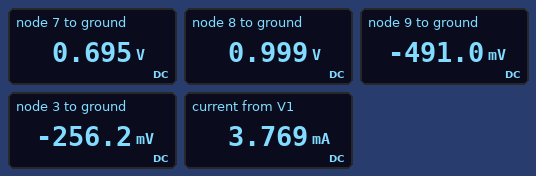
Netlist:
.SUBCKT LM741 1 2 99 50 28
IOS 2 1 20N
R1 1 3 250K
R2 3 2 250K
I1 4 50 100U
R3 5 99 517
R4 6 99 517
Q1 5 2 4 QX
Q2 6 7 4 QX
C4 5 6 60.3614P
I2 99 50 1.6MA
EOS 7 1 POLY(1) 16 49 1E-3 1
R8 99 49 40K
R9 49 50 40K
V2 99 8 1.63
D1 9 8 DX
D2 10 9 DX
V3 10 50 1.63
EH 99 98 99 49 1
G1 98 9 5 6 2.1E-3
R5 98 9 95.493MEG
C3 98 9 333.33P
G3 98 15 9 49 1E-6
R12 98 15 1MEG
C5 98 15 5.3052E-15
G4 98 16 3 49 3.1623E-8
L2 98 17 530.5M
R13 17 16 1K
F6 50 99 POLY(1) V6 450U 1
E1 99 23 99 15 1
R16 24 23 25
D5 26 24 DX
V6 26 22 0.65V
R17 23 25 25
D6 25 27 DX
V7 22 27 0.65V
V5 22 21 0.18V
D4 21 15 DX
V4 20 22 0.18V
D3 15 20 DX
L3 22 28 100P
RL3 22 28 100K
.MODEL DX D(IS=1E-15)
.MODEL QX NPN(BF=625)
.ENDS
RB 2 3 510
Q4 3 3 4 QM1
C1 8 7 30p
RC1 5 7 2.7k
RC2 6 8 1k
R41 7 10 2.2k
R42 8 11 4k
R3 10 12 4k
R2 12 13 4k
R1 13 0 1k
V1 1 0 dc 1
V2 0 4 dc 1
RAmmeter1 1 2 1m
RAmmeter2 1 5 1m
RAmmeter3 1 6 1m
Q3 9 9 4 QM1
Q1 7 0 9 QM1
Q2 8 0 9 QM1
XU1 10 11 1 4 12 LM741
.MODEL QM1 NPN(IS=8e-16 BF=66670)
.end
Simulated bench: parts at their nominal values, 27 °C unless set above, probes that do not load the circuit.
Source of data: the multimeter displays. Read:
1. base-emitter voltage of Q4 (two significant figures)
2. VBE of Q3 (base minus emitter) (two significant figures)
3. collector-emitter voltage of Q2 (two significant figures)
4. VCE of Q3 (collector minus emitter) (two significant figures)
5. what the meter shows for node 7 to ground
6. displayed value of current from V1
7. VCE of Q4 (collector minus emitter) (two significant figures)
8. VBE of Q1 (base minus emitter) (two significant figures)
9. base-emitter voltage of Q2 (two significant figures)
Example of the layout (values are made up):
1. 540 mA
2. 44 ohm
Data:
1. 740 mV
2. 510 mV
3. 1.5 V
4. 510 mV
5. 0.695 V
6. 3.769 mA
7. 740 mV
8. 490 mV
9. 490 mV
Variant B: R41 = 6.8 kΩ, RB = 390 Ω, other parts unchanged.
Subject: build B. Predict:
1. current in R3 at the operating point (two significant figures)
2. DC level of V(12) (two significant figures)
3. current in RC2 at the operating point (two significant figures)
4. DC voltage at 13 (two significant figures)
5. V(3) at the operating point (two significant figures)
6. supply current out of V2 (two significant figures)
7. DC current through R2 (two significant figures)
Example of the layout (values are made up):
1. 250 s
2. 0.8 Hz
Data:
1. 76 µA
2. -16 mV
3. 1.7 µA
4. -3.2 mV
5. -250 mV
6. 4.5 mA
7. 3.2 µA
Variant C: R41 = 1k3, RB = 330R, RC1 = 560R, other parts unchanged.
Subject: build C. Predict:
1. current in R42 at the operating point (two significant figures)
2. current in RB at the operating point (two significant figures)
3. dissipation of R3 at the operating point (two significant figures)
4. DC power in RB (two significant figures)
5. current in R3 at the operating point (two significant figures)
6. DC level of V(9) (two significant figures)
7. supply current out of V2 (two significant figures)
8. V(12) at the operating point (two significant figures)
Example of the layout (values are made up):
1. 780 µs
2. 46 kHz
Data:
1. 810 nA
2. 3.8 mA
3. 120 µW
4. 4.7 mW
5. 170 µA
6. -490 mV
7. 5.1 mA
8. -2.0 mV
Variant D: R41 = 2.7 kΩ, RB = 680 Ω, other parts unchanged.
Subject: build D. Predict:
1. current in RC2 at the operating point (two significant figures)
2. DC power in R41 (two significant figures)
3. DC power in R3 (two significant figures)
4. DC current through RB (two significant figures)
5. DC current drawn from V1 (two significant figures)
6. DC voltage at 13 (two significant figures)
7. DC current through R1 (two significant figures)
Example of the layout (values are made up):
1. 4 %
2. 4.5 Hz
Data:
1. 1.5 µA
2. 31 µW
3. 47 µW
4. 1.9 mA
5. 3.2 mA
6. -2.2 mV
7. 2.2 µA
